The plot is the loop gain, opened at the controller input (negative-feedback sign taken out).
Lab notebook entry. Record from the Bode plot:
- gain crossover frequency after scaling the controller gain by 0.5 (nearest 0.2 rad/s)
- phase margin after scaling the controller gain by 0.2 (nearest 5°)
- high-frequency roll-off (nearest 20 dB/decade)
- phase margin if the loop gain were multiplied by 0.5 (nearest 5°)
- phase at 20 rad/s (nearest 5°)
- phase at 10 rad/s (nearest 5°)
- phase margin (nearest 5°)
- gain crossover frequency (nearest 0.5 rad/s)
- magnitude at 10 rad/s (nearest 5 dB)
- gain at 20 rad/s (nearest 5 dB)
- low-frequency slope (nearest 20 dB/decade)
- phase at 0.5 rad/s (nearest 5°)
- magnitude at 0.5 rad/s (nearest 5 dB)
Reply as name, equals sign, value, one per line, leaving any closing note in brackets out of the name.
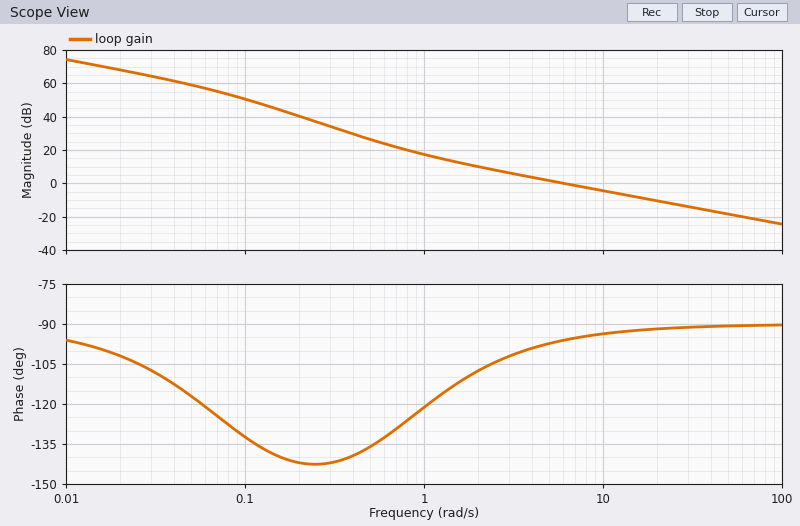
gain crossover frequency after scaling the controller gain by 0.5 = 3.0 rad/s
phase margin after scaling the controller gain by 0.2 = 65°
high-frequency roll-off = -20 dB/decade
phase margin if the loop gain were multiplied by 0.5 = 80°
phase at 20 rad/s = -90°
phase at 10 rad/s = -95°
phase margin = 85°
gain crossover frequency = 6.0 rad/s
magnitude at 10 rad/s = -5 dB
gain at 20 rad/s = -10 dB
low-frequency slope = -20 dB/decade
phase at 0.5 rad/s = -135°
magnitude at 0.5 rad/s = 25 dB
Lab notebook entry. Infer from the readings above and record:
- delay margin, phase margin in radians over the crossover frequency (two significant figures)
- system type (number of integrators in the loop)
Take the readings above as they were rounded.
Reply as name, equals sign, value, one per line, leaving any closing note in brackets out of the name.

delay margin, phase margin in radians over the crossover frequency = 0.25 s
system type = 1
